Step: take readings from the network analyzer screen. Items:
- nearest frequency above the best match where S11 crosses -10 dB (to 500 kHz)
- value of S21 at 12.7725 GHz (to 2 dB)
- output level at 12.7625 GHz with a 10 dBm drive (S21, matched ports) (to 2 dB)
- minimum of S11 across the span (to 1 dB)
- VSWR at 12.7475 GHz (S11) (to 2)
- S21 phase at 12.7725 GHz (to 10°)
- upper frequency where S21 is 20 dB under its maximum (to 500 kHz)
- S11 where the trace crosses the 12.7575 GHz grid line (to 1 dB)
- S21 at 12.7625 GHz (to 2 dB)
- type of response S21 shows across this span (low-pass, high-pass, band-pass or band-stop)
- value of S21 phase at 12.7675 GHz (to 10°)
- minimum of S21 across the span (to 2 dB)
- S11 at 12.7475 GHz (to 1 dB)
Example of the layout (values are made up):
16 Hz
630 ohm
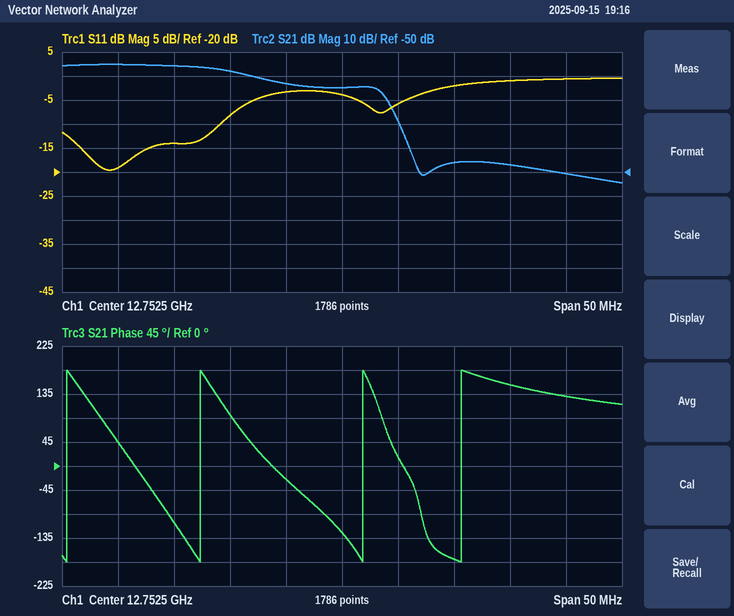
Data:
12.7415 GHz
-50 dB
-36 dBm
-20 dB
6
130°
12.7570 GHz
-6 dB
-46 dB
low-pass
150°
-54 dB
-3 dB
